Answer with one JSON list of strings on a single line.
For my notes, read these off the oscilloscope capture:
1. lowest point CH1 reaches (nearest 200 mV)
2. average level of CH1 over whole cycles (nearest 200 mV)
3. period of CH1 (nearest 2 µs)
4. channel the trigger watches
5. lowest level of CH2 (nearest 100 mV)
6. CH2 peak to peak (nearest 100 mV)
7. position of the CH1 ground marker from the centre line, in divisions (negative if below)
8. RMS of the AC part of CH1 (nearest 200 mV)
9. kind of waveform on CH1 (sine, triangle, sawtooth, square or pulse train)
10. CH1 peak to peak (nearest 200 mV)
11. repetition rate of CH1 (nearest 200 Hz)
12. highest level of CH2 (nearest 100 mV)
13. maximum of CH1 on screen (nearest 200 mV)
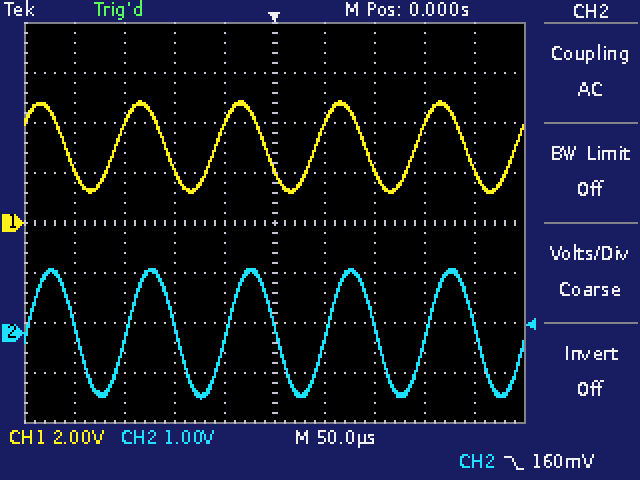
["1.2 V", "3.0 V", "100 µs", "CH2", "-1.3 V", "2.6 V", "0.0 div", "1.2 V", "sine", "3.6 V", "10.0 kHz", "1.3 V", "4.8 V"]
